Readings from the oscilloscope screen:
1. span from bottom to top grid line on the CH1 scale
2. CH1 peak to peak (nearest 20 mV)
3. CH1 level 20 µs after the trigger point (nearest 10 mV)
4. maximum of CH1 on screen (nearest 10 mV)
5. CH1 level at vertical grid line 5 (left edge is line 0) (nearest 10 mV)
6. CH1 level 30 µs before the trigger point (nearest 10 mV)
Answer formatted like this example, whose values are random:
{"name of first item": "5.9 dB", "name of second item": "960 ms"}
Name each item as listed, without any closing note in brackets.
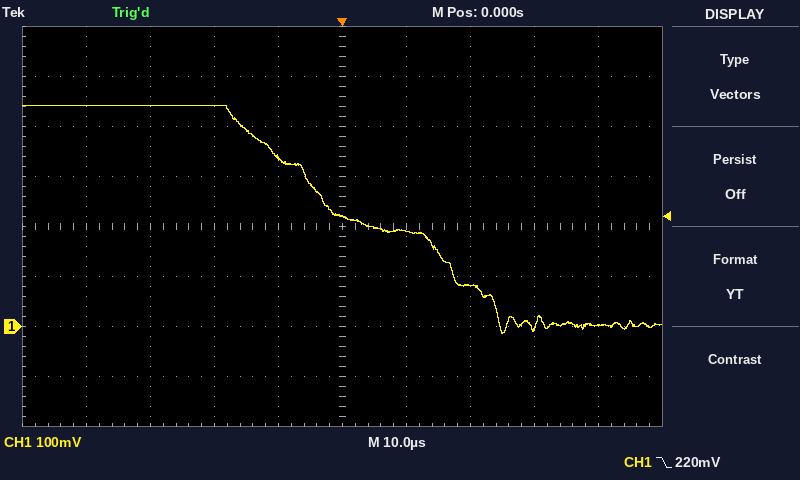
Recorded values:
{"span from bottom to top grid line on the CH1 scale": "800 mV", "CH1 peak to peak": "460 mV", "CH1 level 20 µs after the trigger point": "80 mV", "maximum of CH1 on screen": "440 mV", "CH1 level at vertical grid line 5 (left edge is line 0)": "220 mV", "CH1 level 30 µs before the trigger point": "440 mV"}
